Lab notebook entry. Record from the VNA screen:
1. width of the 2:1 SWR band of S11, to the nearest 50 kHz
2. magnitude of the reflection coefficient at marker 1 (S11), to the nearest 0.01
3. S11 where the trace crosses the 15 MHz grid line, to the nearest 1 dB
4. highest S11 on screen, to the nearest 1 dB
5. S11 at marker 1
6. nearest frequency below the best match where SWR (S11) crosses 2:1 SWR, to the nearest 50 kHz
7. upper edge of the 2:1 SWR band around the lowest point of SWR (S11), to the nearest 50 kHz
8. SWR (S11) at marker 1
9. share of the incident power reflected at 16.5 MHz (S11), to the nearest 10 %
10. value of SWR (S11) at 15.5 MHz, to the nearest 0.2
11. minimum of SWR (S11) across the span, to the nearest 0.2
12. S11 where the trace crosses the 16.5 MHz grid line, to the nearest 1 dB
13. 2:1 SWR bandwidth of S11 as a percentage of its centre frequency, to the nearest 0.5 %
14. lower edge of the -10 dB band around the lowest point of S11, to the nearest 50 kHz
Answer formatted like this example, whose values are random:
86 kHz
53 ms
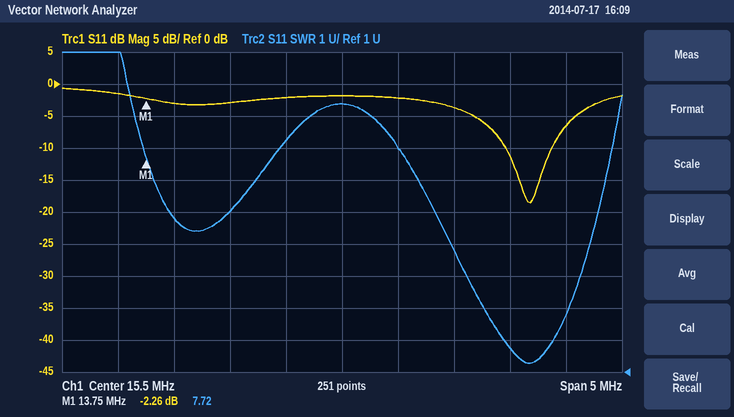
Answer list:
450 kHz
0.77
-2 dB
-1 dB
-2.26 dB
16.95 MHz
17.40 MHz
7.72
40 %
9.4
1.2
-4 dB
2.5 %
16.95 MHz
